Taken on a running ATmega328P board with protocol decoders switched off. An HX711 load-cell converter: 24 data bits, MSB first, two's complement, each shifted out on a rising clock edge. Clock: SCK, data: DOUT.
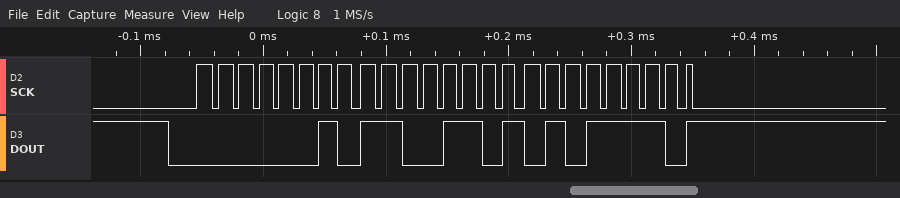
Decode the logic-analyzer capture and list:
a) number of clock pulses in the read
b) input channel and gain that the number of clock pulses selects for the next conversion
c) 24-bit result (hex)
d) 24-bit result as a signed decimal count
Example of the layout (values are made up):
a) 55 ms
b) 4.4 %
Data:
a) 25
b) channel A, gain 128
c) 0x02CD5E
d) 183646
